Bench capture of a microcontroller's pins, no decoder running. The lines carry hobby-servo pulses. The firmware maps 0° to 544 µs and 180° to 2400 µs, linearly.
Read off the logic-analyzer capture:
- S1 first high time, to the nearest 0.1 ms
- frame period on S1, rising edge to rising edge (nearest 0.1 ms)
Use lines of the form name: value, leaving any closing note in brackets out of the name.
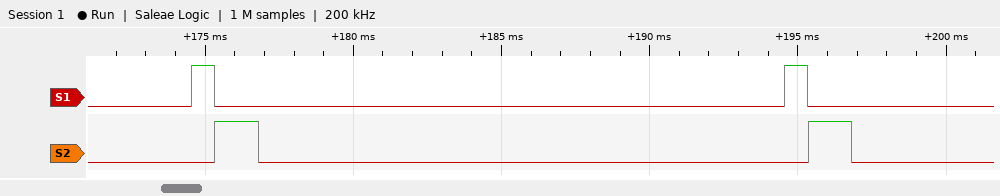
S1 first high time, to the nearest 0.1 ms: 0.8 ms
frame period on S1, rising edge to rising edge: 20.0 ms
